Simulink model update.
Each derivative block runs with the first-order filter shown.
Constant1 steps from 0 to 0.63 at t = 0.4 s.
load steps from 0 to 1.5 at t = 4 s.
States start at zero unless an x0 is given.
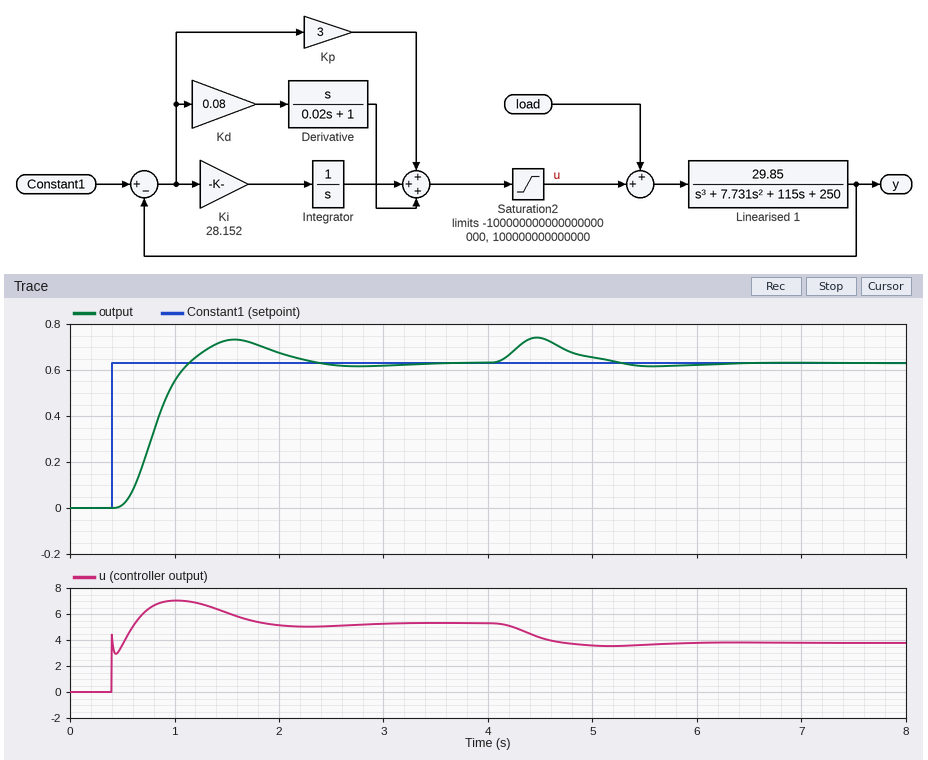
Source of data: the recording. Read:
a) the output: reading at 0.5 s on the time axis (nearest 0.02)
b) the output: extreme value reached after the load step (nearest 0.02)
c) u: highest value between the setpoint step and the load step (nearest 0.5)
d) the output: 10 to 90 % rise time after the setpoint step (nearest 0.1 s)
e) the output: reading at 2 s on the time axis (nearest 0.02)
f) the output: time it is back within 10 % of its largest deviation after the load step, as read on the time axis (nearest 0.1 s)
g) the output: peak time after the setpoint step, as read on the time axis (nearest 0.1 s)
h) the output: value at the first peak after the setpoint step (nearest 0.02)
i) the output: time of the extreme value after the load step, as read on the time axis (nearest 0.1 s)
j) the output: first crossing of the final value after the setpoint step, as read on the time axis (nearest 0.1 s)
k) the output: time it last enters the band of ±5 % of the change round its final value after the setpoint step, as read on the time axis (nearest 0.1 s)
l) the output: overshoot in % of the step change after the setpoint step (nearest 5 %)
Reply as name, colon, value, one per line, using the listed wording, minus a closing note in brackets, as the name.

the output: reading at 0.5 s on the time axis: 0.02
the output: extreme value reached after the load step: 0.74
u: highest value between the setpoint step and the load step: 7.0
the output: 10 to 90 % rise time after the setpoint step: 0.4 s
the output: reading at 2 s on the time axis: 0.68
the output: time it is back within 10 % of its largest deviation after the load step, as read on the time axis: 5.8 s
the output: peak time after the setpoint step, as read on the time axis: 1.6 s
the output: value at the first peak after the setpoint step: 0.74
the output: time of the extreme value after the load step, as read on the time axis: 4.5 s
the output: first crossing of the final value after the setpoint step, as read on the time axis: 1.1 s
the output: time it last enters the band of ±5 % of the change round its final value after the setpoint step, as read on the time axis: 2.1 s
the output: overshoot in % of the step change after the setpoint step: 15 %
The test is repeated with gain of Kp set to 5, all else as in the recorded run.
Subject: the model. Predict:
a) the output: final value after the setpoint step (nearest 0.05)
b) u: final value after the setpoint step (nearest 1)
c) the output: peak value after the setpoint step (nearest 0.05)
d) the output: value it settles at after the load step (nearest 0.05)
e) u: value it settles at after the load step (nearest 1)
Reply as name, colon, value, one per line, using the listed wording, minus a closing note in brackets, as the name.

the output: final value after the setpoint step: 0.65
u: final value after the setpoint step: 5
the output: peak value after the setpoint step: 0.70
the output: value it settles at after the load step: 0.65
u: value it settles at after the load step: 4
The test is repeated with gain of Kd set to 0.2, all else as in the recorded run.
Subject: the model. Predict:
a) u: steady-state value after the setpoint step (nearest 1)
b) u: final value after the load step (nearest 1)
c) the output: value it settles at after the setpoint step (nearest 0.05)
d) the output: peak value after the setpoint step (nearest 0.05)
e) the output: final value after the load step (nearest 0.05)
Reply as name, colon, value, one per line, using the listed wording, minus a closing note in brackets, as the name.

u: steady-state value after the setpoint step: 5
u: final value after the load step: 4
the output: value it settles at after the setpoint step: 0.65
the output: peak value after the setpoint step: 0.75
the output: final value after the load step: 0.65
